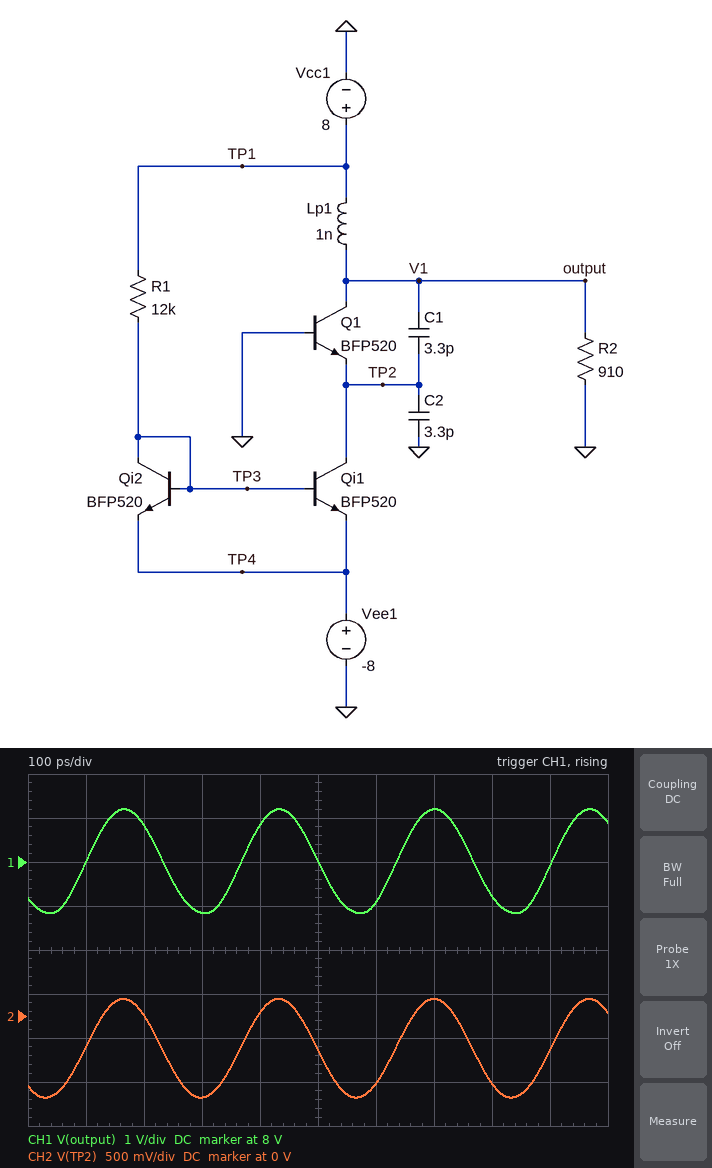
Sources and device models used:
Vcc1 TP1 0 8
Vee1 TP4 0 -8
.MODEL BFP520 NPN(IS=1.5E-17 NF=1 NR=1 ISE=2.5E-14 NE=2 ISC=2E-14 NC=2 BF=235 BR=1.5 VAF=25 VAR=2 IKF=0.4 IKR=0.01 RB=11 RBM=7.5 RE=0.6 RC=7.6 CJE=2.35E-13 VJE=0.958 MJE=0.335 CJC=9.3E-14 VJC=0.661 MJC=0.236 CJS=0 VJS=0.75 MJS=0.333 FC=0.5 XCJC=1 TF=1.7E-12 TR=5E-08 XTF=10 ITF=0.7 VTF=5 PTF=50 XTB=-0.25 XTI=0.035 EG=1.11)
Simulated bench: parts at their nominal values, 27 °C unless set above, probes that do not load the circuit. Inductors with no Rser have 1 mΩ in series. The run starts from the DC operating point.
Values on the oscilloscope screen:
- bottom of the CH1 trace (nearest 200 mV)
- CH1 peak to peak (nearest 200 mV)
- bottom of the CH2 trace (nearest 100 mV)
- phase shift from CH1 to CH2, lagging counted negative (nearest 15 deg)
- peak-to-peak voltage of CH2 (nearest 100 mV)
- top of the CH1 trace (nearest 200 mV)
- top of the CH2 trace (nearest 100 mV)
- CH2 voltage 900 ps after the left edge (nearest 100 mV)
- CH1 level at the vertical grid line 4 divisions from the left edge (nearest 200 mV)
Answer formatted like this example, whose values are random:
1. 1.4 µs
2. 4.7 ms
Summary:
1. 6.8 V
2. 2.4 V
3. -900 mV
4. 0 deg
5. 1.1 V
6. 9.2 V
7. 200 mV
8. -400 mV
9. 8.8 V
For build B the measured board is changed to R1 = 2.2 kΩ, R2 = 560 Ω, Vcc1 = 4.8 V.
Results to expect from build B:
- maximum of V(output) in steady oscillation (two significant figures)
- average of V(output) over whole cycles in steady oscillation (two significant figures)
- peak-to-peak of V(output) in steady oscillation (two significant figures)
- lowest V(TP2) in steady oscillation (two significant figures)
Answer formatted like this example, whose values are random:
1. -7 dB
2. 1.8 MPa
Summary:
1. 8.6 V
2. 4.8 V
3. 7.5 V
4. -1.1 V
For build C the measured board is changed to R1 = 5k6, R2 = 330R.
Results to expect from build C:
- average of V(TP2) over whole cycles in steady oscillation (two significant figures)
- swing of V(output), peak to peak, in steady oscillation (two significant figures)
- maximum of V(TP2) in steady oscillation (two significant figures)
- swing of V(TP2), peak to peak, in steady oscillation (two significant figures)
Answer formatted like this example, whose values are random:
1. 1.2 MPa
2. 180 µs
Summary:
1. -450 mV
2. 2.2 V
3. 69 mV
4. 1.0 V
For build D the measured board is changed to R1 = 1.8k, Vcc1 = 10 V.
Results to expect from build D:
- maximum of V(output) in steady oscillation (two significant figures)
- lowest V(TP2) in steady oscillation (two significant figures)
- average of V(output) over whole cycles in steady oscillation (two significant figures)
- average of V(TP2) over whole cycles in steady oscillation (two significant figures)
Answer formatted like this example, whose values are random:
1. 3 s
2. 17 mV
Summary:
1. 21 V
2. -1.6 V
3. 10 V
4. 3.4 V
